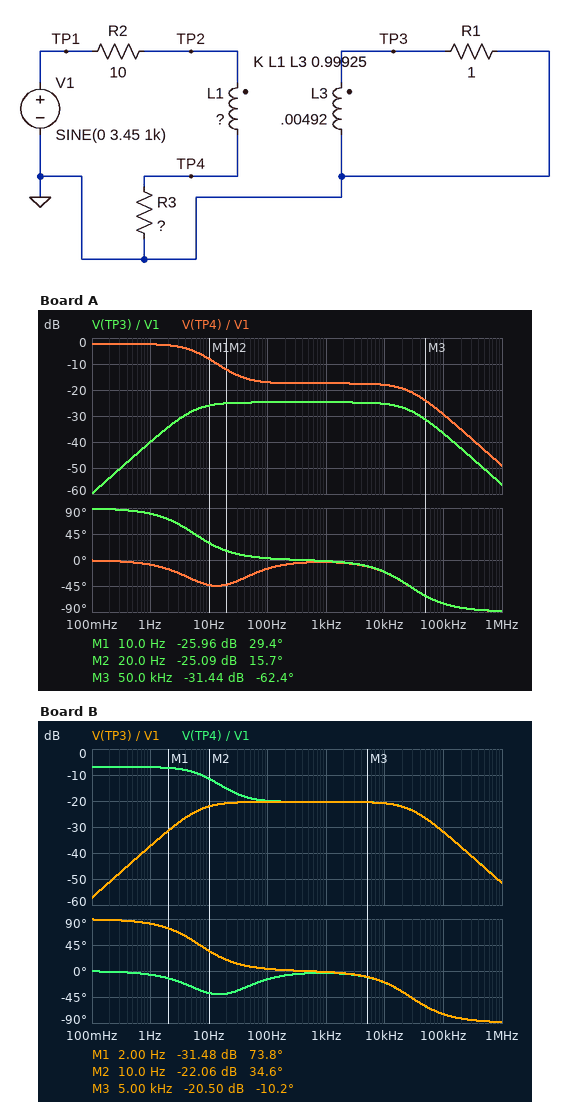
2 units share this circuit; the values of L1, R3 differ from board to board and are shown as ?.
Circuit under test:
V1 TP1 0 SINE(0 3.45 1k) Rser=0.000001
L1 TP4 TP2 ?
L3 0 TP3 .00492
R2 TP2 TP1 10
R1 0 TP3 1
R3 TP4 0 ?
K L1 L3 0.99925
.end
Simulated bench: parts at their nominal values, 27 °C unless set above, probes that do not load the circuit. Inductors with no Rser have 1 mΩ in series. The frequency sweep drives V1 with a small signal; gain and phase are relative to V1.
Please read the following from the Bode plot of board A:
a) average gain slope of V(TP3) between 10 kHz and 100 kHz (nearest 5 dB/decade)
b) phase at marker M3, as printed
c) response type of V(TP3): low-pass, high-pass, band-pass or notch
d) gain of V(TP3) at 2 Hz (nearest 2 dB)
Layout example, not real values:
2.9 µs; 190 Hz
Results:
-10 dB/decade; -62.4 deg; band-pass; -34 dB
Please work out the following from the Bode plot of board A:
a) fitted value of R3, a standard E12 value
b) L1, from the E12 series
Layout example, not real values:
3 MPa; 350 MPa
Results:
33 Ω; 1 H
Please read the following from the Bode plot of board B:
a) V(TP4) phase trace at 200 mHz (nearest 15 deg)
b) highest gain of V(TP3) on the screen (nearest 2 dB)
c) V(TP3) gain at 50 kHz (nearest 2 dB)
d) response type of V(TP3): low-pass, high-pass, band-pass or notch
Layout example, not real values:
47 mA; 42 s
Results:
0 deg; -20 dB; -26 dB; band-pass
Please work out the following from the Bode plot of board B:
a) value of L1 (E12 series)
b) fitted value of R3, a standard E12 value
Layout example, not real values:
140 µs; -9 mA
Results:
330 mH; 8.2 Ω
